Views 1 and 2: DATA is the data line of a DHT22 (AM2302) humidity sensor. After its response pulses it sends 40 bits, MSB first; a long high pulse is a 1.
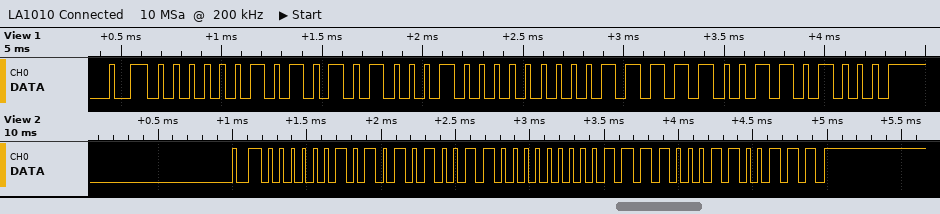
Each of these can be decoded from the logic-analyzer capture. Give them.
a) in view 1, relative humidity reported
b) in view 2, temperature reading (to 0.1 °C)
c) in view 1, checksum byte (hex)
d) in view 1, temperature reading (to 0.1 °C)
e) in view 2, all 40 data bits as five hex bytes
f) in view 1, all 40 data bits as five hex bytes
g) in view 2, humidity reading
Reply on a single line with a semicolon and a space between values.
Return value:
68.0 %; -6.0 °C; 0x68; -6.2 °C; 02 A9 80 3C 67; 02 A8 80 3E 68; 68.1 %
